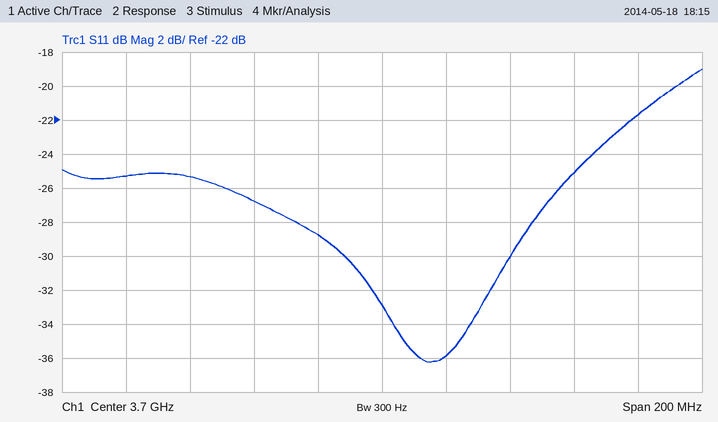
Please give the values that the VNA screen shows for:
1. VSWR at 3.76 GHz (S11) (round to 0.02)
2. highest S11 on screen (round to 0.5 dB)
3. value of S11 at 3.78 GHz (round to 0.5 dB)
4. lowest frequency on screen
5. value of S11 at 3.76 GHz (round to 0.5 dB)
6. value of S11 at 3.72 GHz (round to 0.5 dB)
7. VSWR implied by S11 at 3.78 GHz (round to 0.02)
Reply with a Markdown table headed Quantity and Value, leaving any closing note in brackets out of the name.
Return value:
| Quantity | Value |
|---|---|
| VSWR at 3.76 GHz (S11) | 1.12 |
| highest S11 on screen | -19.0 dB |
| value of S11 at 3.78 GHz | -21.5 dB |
| lowest frequency on screen | 3.6 GHz |
| value of S11 at 3.76 GHz | -25.0 dB |
| value of S11 at 3.72 GHz | -36.0 dB |
| VSWR implied by S11 at 3.78 GHz | 1.18 |
